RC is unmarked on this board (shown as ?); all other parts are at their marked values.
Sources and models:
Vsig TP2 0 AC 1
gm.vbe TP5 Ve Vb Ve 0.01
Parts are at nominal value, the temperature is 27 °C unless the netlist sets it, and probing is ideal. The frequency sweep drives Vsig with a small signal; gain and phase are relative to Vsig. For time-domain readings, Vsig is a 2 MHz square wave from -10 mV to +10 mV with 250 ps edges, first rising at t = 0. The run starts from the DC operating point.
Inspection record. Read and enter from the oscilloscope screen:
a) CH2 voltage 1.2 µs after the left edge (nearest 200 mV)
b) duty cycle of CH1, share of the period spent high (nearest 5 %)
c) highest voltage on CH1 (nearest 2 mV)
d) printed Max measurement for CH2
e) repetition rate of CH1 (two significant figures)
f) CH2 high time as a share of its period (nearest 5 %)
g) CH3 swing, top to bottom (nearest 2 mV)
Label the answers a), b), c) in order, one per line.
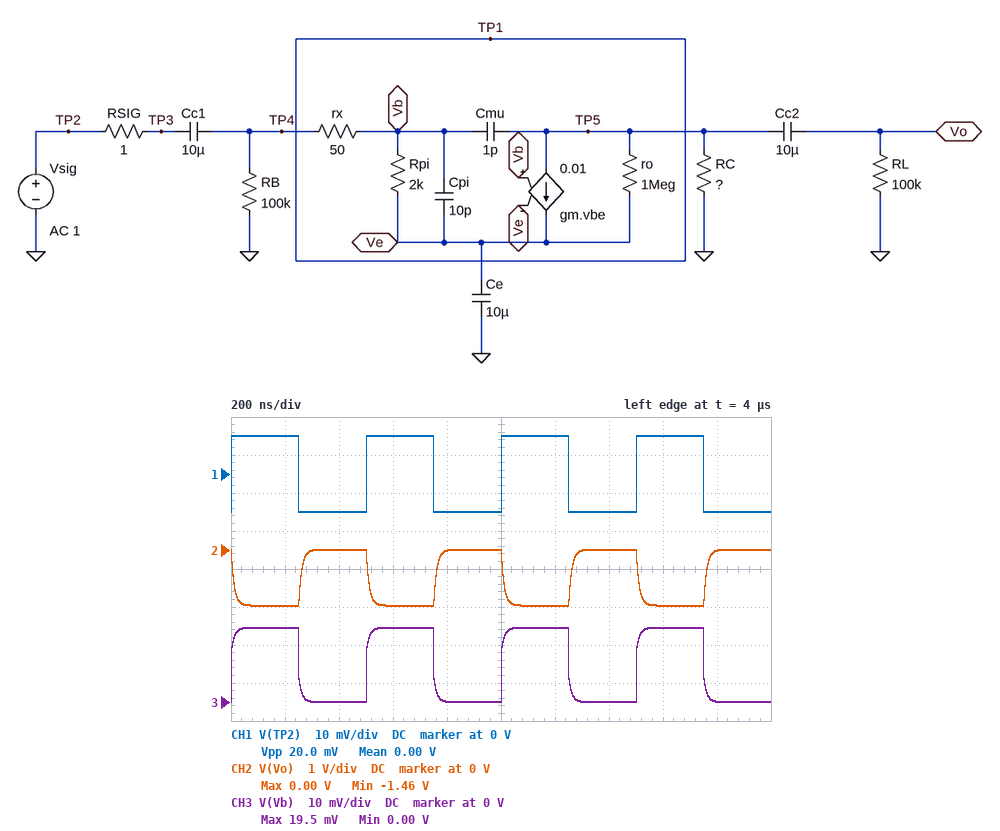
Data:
a) -1.4 V
b) 50 %
c) 10 mV
d) 0.00 V
e) 2.0 MHz
f) 50 %
g) 20 mV
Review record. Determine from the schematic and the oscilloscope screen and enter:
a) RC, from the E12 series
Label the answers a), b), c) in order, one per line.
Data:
a) 8.2 kΩ
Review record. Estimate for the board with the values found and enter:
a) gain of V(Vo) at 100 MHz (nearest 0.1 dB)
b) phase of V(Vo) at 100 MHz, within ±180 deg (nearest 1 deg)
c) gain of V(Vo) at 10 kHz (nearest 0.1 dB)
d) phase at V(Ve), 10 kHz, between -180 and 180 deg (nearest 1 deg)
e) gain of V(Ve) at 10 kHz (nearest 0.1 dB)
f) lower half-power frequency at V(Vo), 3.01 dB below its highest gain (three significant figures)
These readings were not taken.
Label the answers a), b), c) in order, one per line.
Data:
a) 19.9 dB
b) 83 deg
c) 37.3 dB
d) -89 deg
e) -35.8 dB
f) 170 Hz
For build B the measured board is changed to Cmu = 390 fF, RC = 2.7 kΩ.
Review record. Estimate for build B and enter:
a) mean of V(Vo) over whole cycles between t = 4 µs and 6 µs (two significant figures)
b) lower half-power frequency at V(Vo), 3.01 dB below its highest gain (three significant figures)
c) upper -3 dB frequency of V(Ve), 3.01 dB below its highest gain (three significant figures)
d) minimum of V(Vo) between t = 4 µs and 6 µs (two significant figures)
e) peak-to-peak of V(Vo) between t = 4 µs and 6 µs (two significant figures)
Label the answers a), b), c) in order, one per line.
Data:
a) -250 mV
b) 170 Hz
c) 171 Hz
d) -510 mV
e) 510 mV
